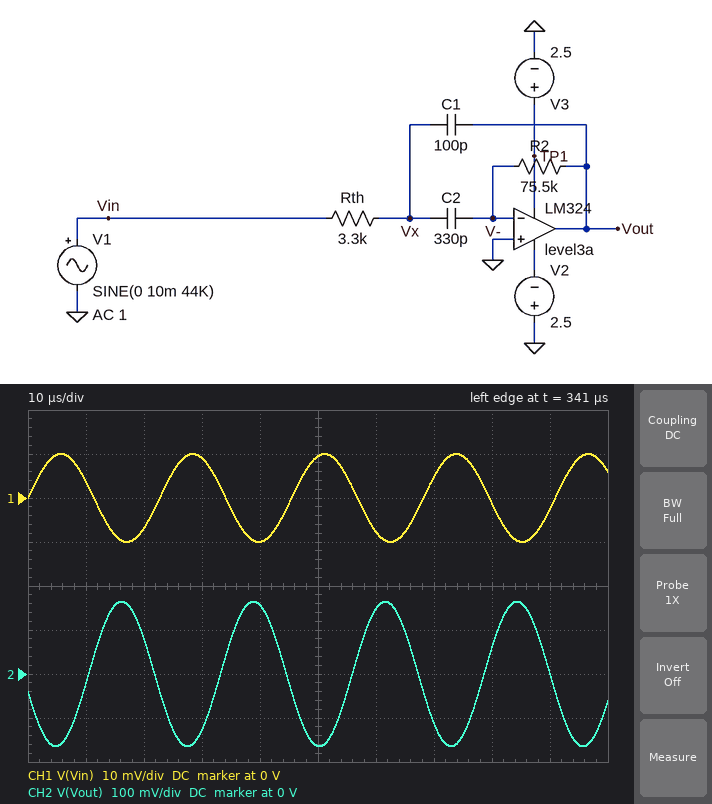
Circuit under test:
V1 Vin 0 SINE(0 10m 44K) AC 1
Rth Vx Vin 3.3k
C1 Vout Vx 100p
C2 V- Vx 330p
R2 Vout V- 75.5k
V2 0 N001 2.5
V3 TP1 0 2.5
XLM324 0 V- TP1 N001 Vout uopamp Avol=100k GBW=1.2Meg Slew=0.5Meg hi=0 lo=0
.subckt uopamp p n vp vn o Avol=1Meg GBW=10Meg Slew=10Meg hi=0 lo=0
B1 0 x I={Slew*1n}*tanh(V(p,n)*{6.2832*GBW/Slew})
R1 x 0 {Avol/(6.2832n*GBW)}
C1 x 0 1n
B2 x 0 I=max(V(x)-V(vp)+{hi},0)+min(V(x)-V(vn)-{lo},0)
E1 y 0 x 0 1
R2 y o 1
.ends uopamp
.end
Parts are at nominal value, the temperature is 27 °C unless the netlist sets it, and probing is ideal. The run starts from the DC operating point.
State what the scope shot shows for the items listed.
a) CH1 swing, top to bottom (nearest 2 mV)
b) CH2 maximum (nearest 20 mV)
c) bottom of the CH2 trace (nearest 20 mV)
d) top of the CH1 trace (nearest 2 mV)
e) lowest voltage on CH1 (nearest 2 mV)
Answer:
20 mV
160 mV
-160 mV
10 mV
-10 mV
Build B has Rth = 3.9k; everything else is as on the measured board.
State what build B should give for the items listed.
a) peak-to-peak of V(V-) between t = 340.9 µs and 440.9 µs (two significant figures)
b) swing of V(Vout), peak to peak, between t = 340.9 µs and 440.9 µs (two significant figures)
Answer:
11 mV
290 mV
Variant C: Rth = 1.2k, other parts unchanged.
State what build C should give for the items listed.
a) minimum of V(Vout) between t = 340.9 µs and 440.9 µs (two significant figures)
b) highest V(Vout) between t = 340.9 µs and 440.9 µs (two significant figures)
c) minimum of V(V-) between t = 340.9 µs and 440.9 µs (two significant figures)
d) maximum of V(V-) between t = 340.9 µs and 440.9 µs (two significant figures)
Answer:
-130 mV
130 mV
-4.7 mV
4.7 mV
